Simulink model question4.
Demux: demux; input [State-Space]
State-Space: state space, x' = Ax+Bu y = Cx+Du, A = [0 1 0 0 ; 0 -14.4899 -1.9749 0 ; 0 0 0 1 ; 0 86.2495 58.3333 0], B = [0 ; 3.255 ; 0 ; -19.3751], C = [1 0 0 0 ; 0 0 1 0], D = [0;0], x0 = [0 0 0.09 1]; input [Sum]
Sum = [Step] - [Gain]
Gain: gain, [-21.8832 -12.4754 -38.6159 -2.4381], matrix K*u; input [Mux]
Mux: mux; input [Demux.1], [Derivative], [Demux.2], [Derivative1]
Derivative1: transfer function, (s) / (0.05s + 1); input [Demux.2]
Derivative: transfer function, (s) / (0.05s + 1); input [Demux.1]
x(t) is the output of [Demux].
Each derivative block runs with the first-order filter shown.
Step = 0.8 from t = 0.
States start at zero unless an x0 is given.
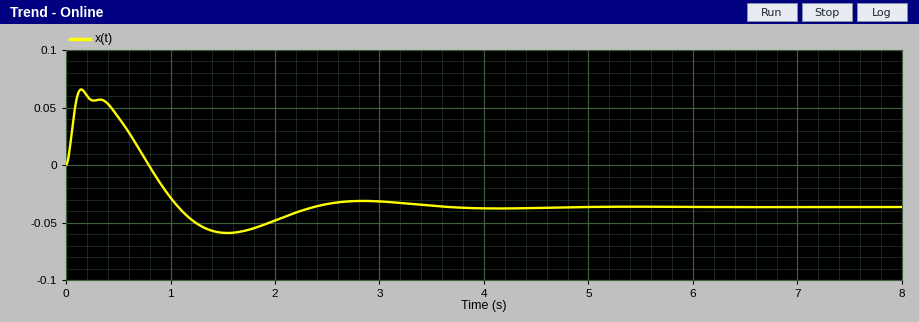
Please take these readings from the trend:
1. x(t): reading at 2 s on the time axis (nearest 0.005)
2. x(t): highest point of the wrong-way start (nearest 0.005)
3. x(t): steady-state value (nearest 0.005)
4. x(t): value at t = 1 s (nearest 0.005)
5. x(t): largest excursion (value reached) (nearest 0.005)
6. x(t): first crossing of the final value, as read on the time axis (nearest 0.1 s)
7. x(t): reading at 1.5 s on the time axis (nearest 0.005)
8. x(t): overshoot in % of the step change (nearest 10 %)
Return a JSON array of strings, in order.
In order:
["-0.050", "0.065", "-0.035", "-0.030", "-0.060", "1.1 s", "-0.060", "60 %"]
